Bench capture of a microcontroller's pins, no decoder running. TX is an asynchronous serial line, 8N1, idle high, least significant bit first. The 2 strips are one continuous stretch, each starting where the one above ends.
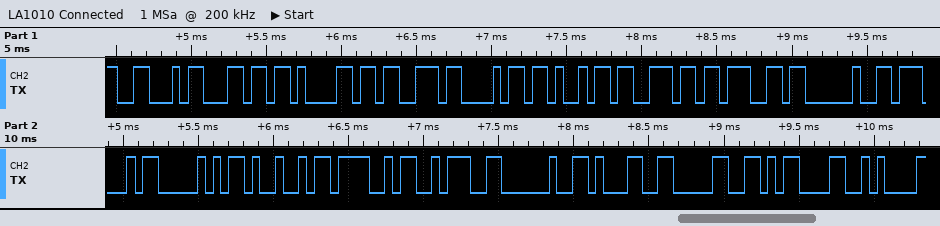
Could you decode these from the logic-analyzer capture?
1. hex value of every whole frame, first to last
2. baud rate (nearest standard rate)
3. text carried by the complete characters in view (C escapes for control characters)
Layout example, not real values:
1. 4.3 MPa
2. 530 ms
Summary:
1. 0x46 0x6C 0x61 0x73 0x68 0x69 0x6E 0x67 0x20 0x47 0x50 0x49 0x4F 0x3A 0x20 0x31 0x30 0x0D 0x0A
2. 19200 baud
3. "Flashing GPIO: 10\r\n"
